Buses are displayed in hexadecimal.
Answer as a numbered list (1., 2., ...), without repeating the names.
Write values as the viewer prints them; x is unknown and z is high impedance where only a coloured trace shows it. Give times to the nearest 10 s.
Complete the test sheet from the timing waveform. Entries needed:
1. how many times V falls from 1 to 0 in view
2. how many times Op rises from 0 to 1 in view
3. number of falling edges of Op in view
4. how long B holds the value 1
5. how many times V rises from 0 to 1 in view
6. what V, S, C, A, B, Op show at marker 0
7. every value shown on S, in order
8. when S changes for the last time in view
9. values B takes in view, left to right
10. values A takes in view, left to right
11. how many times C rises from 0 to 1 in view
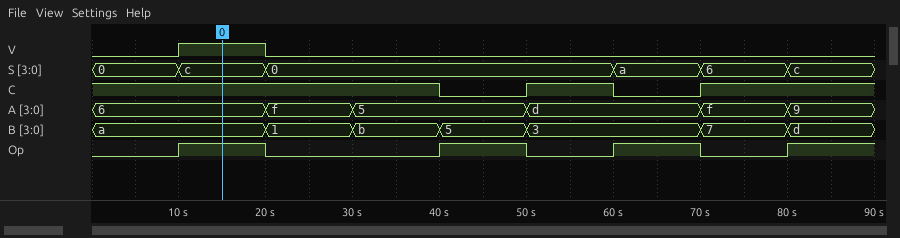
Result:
1. 1
2. 4
3. 3
4. 10 s
5. 1
6. V=1, S=c, C=1, A=6, B=a, Op=1
7. 0, c, 0, a, 6, c
8. 80 s
9. a, 1, b, 5, 3, 7, d
10. 6, f, 5, d, f, 9
11. 2
